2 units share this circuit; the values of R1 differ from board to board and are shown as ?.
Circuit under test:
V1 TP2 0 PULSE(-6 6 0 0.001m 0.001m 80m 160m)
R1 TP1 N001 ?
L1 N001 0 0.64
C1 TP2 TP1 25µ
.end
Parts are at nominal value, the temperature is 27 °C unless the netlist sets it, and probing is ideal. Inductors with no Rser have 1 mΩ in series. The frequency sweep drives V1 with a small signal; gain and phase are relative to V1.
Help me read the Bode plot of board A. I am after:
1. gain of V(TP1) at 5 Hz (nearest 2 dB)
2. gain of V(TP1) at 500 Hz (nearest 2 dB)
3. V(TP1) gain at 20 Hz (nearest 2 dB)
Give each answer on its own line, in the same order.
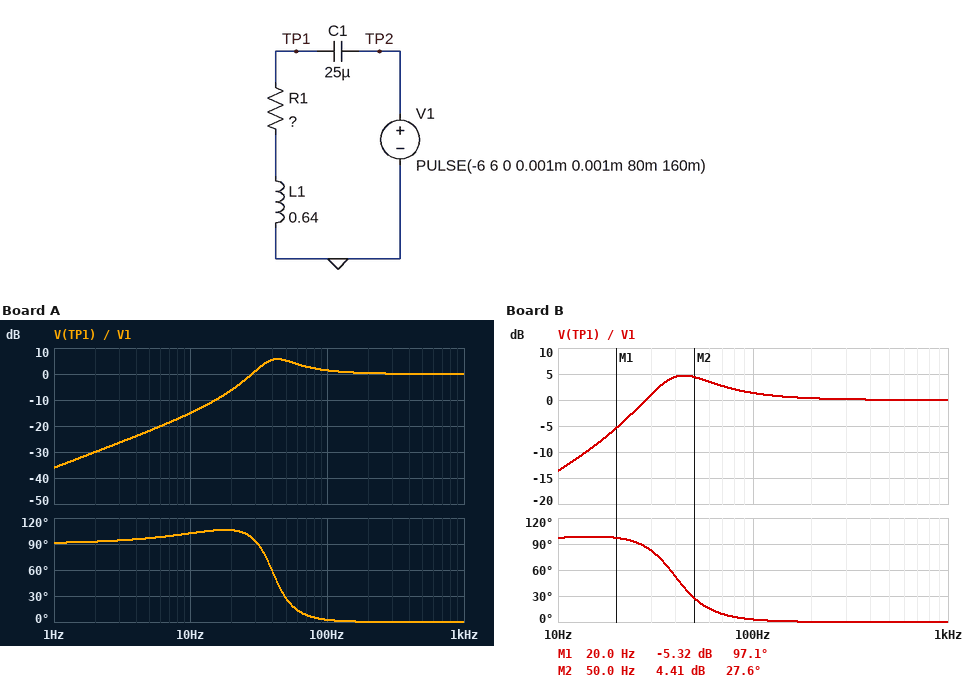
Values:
-22 dB
0 dB
-6 dB
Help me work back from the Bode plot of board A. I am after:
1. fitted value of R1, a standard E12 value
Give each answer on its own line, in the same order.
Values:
100 Ω
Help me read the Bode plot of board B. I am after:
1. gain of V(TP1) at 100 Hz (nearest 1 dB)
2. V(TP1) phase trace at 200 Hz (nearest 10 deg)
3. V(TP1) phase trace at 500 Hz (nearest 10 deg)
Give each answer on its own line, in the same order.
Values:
1 dB
0 deg
0 deg
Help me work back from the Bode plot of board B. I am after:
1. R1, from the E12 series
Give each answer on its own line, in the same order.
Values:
120 Ω
